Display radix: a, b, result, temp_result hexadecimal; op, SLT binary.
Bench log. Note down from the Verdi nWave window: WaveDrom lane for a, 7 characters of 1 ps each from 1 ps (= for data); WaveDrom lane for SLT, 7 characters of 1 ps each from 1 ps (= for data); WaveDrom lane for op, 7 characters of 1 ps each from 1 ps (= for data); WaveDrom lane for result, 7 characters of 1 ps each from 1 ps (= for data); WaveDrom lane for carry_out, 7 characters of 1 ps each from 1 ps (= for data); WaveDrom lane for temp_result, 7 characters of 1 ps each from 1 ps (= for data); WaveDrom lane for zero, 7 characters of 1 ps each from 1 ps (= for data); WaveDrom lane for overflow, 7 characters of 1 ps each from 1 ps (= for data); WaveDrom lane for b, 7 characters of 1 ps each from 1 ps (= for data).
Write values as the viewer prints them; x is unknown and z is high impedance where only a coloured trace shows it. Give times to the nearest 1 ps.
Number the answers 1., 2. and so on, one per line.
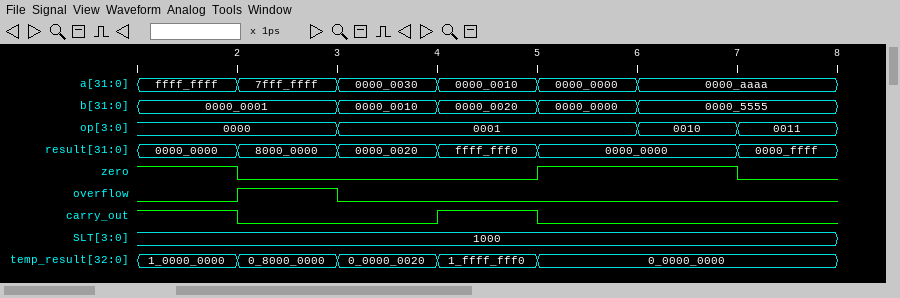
1. {name: 'a', wave: '======.', data: 'ffff_ffff 7fff_ffff 0000_0030 0000_0010 0000_0000 0000_aaaa'}
2. {name: 'SLT', wave: '=......', data: '1000'}
3. {name: 'op', wave: '=.=..==', data: '0000 0001 0010 0011'}
4. {name: 'result', wave: '=====.=', data: '0000_0000 8000_0000 0000_0020 ffff_fff0 0000_0000 0000_ffff'}
5. {name: 'carry_out', wave: '10.10..'}
6. {name: 'temp_result', wave: '=====..', data: '1_0000_0000 0_8000_0000 0_0000_0020 1_ffff_fff0 0_0000_0000'}
7. {name: 'zero', wave: '10..1.0'}
8. {name: 'overflow', wave: '010....'}
9. {name: 'b', wave: '=.====.', data: '0000_0001 0000_0010 0000_0020 0000_0000 0000_5555'}
